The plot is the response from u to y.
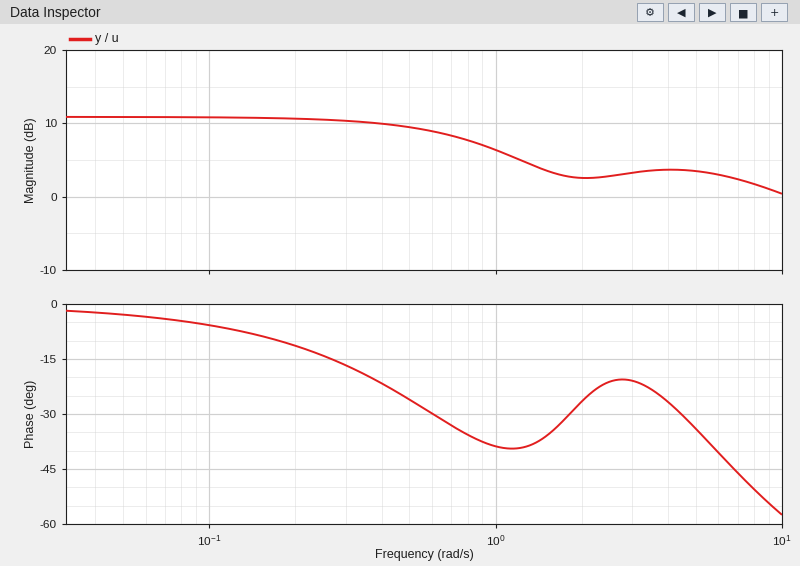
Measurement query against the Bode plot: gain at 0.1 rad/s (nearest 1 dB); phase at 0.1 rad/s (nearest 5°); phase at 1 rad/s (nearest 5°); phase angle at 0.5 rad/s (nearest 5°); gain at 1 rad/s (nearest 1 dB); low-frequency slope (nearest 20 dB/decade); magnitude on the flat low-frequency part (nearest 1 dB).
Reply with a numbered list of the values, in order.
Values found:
1. 11 dB
2. -5°
3. -40°
4. -25°
5. 6 dB
6. 0 dB/decade
7. 11 dB
